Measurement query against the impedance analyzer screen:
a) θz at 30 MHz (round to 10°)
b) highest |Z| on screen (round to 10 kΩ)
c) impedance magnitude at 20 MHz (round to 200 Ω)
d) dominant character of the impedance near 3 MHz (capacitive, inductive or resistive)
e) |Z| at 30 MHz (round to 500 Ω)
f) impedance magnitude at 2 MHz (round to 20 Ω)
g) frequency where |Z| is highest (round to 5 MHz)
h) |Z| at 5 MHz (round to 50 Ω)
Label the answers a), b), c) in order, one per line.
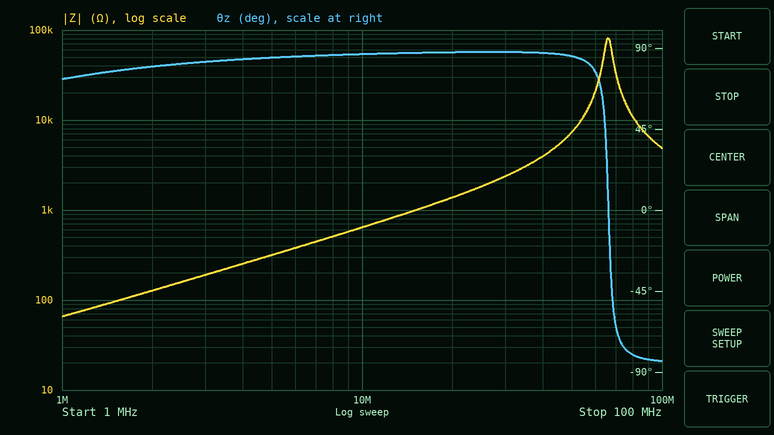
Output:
a) 90°
b) 80 kΩ
c) 1.4 kΩ
d) inductive
e) 2.5 kΩ
f) 120 Ω
g) 65 MHz
h) 300 Ω
